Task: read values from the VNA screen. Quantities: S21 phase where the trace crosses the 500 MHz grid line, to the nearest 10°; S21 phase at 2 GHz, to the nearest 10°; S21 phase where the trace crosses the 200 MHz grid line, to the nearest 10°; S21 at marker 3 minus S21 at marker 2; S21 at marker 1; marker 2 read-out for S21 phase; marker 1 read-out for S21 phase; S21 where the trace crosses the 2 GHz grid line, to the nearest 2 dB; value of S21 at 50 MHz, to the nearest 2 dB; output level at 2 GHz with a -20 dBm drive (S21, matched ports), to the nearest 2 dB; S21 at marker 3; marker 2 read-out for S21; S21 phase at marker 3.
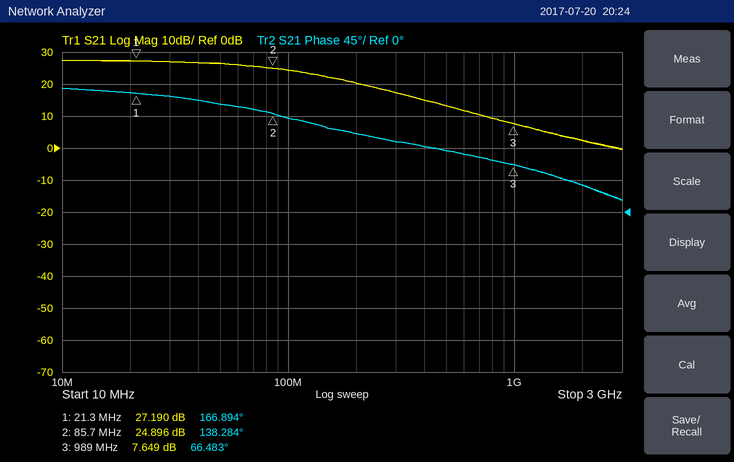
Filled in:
90°
40°
110°
-17.247 dB
27.190 dB
138.284°
166.894°
2 dB
26 dB
-18 dBm
7.649 dB
24.896 dB
66.483°
